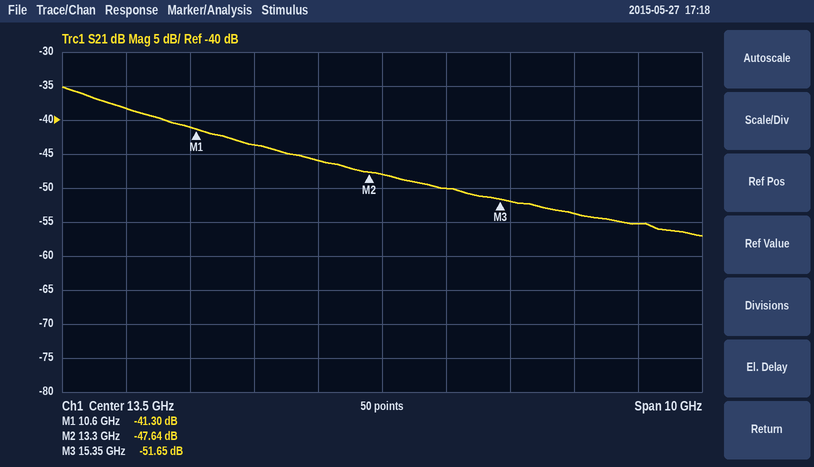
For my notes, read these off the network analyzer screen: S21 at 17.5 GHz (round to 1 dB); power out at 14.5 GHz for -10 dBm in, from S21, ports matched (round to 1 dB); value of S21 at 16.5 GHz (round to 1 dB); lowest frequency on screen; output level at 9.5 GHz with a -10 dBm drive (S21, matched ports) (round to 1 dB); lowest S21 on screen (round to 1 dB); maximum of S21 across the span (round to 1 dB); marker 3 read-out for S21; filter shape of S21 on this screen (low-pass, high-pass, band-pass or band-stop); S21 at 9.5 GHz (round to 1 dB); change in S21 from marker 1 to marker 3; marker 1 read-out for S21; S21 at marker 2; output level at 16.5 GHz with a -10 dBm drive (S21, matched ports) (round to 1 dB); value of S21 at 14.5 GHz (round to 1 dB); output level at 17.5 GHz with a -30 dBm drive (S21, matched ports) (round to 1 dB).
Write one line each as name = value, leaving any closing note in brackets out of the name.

S21 at 17.5 GHz = -55 dB
power out at 14.5 GHz for -10 dBm in, from S21, ports matched = -60 dBm
value of S21 at 16.5 GHz = -54 dB
lowest frequency on screen = 8.5 GHz
output level at 9.5 GHz with a -10 dBm drive (S21, matched ports) = -48 dBm
lowest S21 on screen = -57 dB
maximum of S21 across the span = -35 dB
marker 3 read-out for S21 = -51.65 dB
filter shape of S21 on this screen = low-pass
S21 at 9.5 GHz = -38 dB
change in S21 from marker 1 to marker 3 = -10.35 dB
marker 1 read-out for S21 = -41.30 dB
S21 at marker 2 = -47.64 dB
output level at 16.5 GHz with a -10 dBm drive (S21, matched ports) = -64 dBm
value of S21 at 14.5 GHz = -50 dB
output level at 17.5 GHz with a -30 dBm drive (S21, matched ports) = -85 dBm
